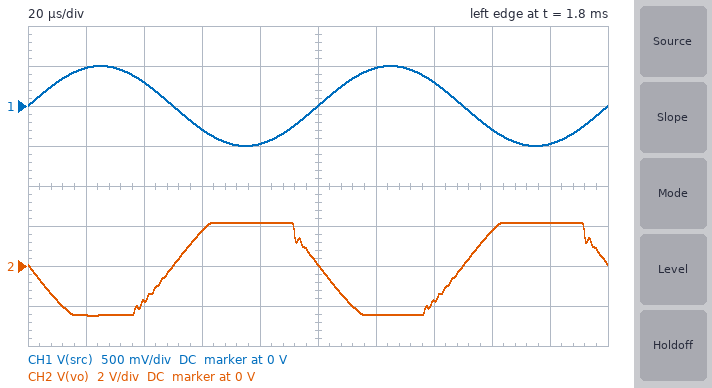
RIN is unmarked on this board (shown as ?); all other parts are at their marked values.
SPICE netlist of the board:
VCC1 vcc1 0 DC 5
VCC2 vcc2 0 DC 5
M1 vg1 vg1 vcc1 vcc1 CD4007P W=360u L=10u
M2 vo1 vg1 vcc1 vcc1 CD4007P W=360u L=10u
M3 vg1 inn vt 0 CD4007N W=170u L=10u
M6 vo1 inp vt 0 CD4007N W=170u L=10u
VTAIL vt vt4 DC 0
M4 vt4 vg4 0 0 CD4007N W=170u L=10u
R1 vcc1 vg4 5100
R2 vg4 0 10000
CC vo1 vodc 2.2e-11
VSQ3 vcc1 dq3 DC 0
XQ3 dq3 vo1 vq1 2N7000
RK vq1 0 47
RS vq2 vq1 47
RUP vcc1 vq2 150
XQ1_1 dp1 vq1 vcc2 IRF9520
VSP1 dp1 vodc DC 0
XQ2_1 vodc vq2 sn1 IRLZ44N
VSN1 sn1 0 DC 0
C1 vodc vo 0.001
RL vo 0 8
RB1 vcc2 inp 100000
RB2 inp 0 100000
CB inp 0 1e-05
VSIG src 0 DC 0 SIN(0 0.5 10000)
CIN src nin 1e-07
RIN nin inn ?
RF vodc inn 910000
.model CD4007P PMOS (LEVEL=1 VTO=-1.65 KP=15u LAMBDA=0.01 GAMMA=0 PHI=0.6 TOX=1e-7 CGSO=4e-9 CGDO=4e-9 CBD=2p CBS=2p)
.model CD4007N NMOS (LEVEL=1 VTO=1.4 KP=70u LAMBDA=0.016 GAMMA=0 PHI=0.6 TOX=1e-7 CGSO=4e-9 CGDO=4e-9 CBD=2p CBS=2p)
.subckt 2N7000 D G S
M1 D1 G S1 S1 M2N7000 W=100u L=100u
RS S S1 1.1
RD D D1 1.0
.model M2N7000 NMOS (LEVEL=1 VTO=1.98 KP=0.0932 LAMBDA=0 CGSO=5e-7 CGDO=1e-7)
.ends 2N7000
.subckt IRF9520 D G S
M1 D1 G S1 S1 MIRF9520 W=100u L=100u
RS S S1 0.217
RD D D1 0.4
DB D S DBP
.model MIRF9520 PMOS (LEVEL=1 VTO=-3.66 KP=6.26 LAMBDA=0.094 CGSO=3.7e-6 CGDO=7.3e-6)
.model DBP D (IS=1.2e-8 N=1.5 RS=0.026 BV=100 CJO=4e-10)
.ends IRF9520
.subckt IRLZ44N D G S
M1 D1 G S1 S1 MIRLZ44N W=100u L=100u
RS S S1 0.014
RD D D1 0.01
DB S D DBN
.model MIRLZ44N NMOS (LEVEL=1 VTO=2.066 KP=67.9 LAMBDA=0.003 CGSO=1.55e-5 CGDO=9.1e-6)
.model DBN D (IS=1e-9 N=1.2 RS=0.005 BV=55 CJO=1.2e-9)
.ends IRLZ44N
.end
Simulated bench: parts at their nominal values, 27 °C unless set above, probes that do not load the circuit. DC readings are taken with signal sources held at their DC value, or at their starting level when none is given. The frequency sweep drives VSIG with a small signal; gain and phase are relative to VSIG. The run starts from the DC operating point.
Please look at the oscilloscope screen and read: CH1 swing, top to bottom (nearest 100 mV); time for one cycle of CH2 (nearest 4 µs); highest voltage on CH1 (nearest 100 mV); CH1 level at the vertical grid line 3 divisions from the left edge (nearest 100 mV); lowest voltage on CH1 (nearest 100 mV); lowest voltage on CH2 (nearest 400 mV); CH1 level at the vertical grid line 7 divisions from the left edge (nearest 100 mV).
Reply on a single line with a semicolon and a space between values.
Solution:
1.0 V; 100 µs; 500 mV; -300 mV; -500 mV; -2.4 V; 300 mV
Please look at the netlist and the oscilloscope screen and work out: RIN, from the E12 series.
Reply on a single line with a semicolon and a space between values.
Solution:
150 kΩ
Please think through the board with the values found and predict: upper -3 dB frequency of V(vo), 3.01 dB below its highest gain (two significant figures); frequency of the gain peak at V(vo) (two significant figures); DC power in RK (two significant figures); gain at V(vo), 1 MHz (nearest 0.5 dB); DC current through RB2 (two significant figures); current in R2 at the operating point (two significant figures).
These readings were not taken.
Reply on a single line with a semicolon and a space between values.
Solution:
510 kHz; 470 kHz; 31 mW; 2.0 dB; 25 µA; 330 µA
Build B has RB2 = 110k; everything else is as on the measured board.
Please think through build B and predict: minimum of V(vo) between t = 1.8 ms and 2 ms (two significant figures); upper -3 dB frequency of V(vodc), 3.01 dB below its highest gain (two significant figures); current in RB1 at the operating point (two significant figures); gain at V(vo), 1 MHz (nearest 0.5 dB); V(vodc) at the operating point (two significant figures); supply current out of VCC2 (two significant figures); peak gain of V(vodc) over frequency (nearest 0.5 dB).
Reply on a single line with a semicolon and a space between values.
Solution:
-2.6 V; 520 kHz; 24 µA; 3.0 dB; 2.6 V; 59 mA; 32.0 dB
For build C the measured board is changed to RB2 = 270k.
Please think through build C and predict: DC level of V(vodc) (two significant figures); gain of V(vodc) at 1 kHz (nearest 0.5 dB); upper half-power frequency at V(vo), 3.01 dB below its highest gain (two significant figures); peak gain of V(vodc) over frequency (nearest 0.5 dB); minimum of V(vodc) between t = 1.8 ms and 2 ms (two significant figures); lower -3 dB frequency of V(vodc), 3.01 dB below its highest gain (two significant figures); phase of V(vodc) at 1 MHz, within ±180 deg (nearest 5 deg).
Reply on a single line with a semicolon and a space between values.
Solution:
4.3 V; 11.5 dB; 210 kHz; 13.0 dB; 2.4 V; 6.3 Hz; -10 deg
